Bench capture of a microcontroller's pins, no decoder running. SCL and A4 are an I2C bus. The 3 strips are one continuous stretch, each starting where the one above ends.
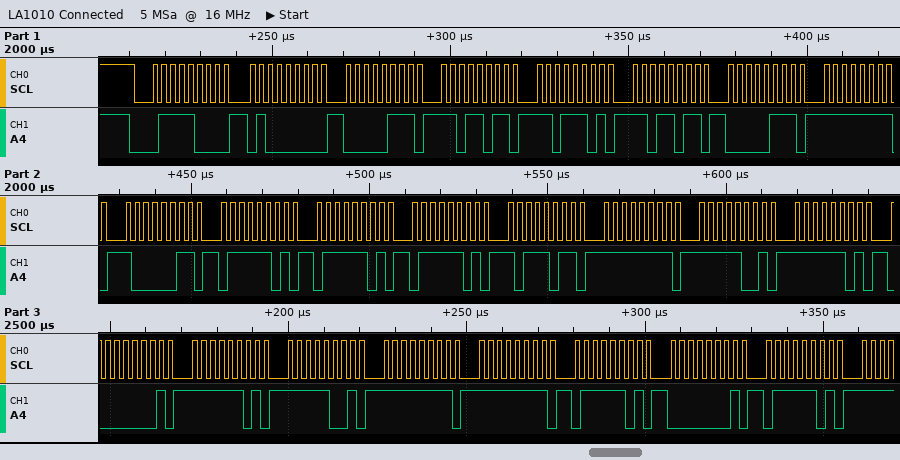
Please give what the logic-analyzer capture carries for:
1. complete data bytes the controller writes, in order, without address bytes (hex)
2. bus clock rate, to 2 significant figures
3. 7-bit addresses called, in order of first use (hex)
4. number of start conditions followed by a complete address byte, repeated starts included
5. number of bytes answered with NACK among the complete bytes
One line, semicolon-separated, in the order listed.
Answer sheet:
40 07 DB DD DB 07 FF 83 7D 7D 7D BB FF F9 FD 01 FD F9 FF FF 7D 01 7D; 400 kHz; 0x3C; 1; 0
